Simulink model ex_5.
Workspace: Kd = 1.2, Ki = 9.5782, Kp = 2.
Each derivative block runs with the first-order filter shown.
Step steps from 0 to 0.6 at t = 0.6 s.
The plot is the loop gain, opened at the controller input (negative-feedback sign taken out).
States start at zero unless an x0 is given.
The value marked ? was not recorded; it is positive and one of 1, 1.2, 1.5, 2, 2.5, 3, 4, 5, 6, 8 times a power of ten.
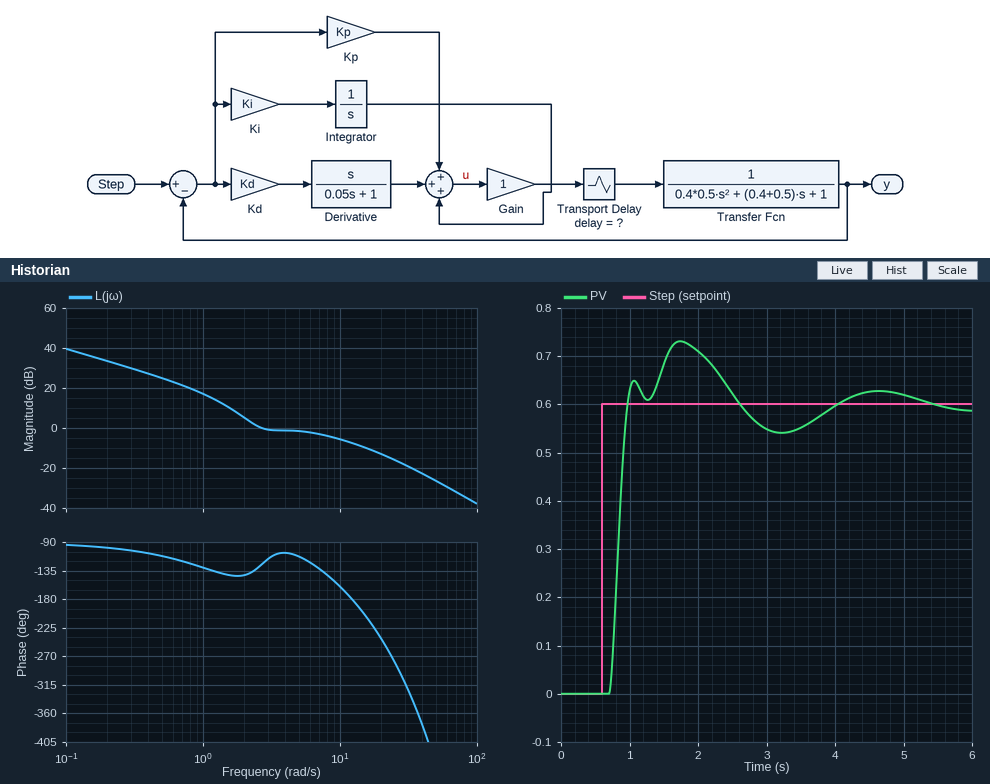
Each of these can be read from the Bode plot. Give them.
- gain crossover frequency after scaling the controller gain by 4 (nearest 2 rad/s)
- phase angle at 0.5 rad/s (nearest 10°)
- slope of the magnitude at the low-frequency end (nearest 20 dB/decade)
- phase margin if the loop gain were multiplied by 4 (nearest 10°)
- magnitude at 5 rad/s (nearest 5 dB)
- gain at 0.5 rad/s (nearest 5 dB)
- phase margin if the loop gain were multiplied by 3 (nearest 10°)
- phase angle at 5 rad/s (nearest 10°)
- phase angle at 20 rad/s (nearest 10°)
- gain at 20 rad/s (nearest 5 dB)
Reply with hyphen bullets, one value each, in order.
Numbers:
- 18 rad/s
- -110°
- -20 dB/decade
- -50°
- 0 dB
- 25 dB
- -20°
- -110°
- -240°
- -15 dB
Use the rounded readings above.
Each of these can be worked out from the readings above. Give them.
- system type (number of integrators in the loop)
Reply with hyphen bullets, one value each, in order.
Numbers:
- 1
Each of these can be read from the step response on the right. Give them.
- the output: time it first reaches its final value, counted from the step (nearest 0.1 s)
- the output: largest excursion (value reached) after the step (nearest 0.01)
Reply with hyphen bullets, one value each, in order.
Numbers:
- 0.4 s
- 0.73
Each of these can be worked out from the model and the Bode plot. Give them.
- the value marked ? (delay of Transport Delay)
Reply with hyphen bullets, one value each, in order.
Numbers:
- 0.1
